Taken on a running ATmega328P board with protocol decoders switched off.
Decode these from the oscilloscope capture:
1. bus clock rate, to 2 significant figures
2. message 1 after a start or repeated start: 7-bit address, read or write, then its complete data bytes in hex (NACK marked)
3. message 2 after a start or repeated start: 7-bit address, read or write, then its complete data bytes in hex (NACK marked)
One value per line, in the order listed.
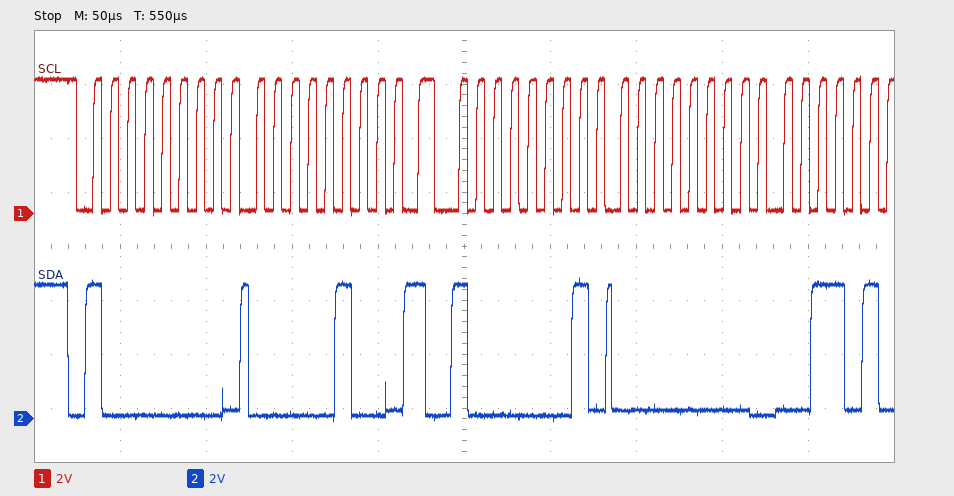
100 kHz
0x40 write: 04
0x40 read: 00
